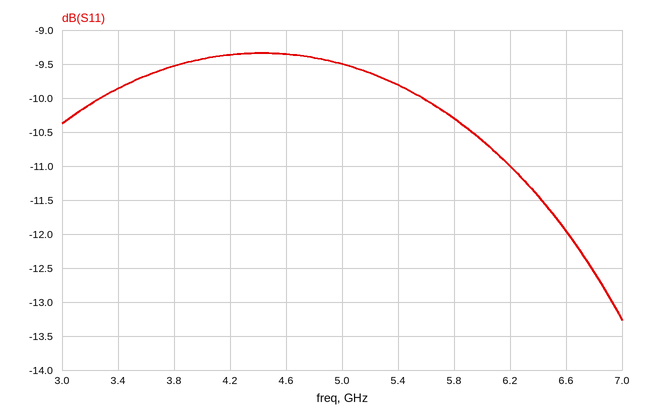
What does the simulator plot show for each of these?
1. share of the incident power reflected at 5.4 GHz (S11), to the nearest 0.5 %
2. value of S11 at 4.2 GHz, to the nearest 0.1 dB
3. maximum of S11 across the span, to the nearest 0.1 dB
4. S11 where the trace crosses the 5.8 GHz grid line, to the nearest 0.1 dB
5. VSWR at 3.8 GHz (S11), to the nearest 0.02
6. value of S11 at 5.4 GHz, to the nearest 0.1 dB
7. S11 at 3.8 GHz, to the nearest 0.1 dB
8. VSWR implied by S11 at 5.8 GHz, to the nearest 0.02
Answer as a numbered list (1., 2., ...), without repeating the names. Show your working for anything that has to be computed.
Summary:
1. 10^(-9.8/10) ≈ 10.5 %
2. -9.4 dB
3. -9.3 dB
4. -10.3 dB
5. |Γ| = 10^(-9.5/20) = 0.3350; VSWR = (1 + 0.3350)/(1 − 0.3350) ≈ 2.01, so 2.00 to the nearest 0.02
6. -9.8 dB
7. -9.5 dB
8. |Γ| = 10^(-10.3/20) = 0.3055; VSWR = (1 + 0.3055)/(1 − 0.3055) ≈ 1.88
